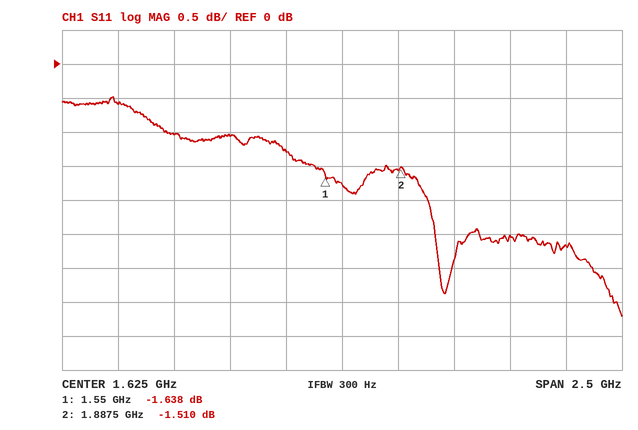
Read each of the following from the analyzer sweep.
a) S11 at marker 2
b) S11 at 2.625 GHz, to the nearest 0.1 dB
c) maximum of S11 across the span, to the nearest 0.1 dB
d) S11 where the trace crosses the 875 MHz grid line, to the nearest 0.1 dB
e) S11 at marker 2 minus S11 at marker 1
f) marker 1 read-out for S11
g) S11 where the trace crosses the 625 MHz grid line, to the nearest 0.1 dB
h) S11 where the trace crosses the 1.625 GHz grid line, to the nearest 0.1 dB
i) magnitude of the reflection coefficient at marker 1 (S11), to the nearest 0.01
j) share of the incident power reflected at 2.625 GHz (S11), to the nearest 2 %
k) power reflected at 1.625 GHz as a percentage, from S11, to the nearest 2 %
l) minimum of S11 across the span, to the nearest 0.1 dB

-1.510 dB
-2.7 dB
-0.5 dB
-1.0 dB
0.128 dB
-1.638 dB
-0.6 dB
-1.8 dB
0.83
54 %
66 %
-3.7 dB
